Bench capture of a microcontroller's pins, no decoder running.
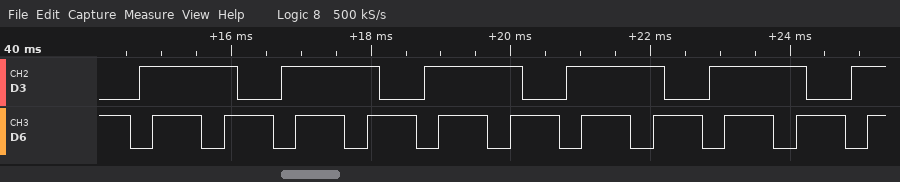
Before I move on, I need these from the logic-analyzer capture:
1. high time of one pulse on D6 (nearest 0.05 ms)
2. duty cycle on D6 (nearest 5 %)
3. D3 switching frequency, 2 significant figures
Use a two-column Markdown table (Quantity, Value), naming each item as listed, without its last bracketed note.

| Quantity | Value |
|---|---|
| high time of one pulse on D6 | 0.70 ms |
| duty cycle on D6 | 70 % |
| D3 switching frequency, 2 significant figures | 490 Hz |
